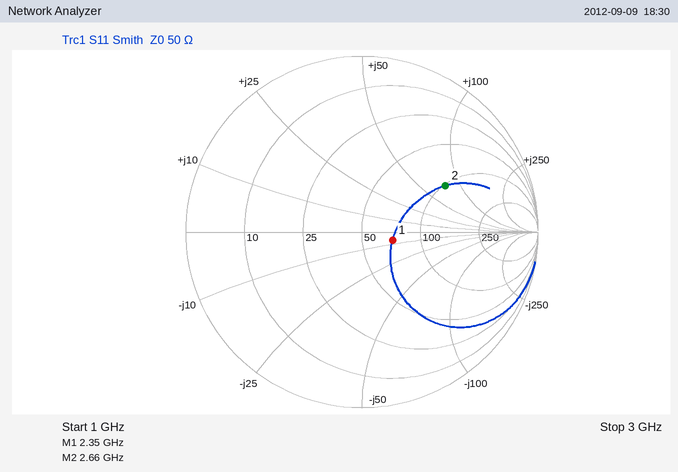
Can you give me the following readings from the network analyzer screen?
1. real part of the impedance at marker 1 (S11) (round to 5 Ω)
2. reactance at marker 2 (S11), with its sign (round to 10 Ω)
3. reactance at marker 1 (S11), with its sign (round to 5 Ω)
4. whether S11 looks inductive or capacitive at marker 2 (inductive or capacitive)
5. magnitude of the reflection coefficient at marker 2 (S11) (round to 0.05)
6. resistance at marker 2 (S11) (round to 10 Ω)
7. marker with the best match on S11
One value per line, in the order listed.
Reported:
70 Ω
+80 Ω
-5 Ω
inductive
0.55
100 Ω
marker 1
